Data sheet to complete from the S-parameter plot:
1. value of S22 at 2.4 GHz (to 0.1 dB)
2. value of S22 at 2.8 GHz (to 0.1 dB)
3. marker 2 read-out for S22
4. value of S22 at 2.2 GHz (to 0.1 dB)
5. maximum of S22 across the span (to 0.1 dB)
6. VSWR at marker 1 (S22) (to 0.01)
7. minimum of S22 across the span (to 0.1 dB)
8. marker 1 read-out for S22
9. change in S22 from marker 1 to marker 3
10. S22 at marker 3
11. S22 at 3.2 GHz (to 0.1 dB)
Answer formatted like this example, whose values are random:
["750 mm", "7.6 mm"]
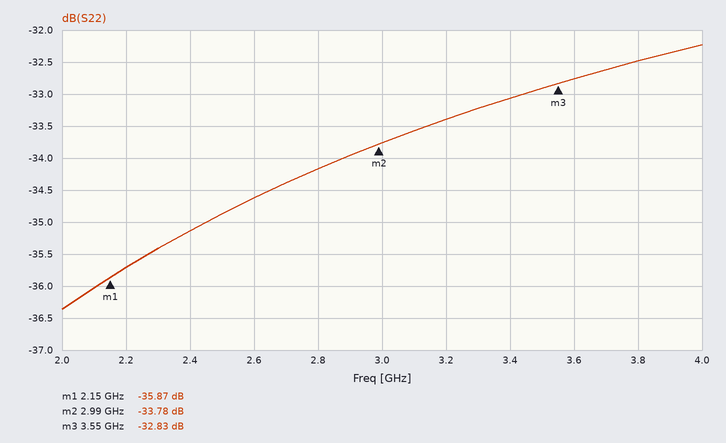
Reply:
["-35.1 dB", "-34.2 dB", "-33.78 dB", "-35.7 dB", "-32.2 dB", "1.03", "-36.4 dB", "-35.87 dB", "3.04 dB", "-32.83 dB", "-33.4 dB"]
